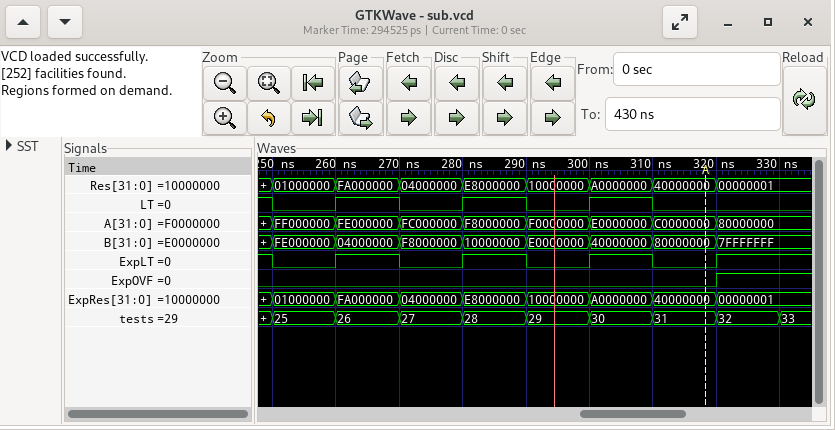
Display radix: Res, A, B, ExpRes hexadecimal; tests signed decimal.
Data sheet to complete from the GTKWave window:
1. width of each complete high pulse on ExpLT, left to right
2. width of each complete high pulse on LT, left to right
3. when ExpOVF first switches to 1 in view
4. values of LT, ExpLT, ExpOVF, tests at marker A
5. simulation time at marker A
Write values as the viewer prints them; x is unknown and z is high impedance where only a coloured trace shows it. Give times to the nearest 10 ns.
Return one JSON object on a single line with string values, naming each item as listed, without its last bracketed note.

{"width of each complete high pulse on ExpLT, left to right": "10 ns, 10 ns, 10 ns", "width of each complete high pulse on LT, left to right": "10 ns, 10 ns, 10 ns", "when ExpOVF first switches to 1 in view": "320 ns", "values of LT, ExpLT, ExpOVF, tests at marker A": "LT=0, ExpLT=0, ExpOVF=0, tests=31", "simulation time at marker A": "320 ns"}
